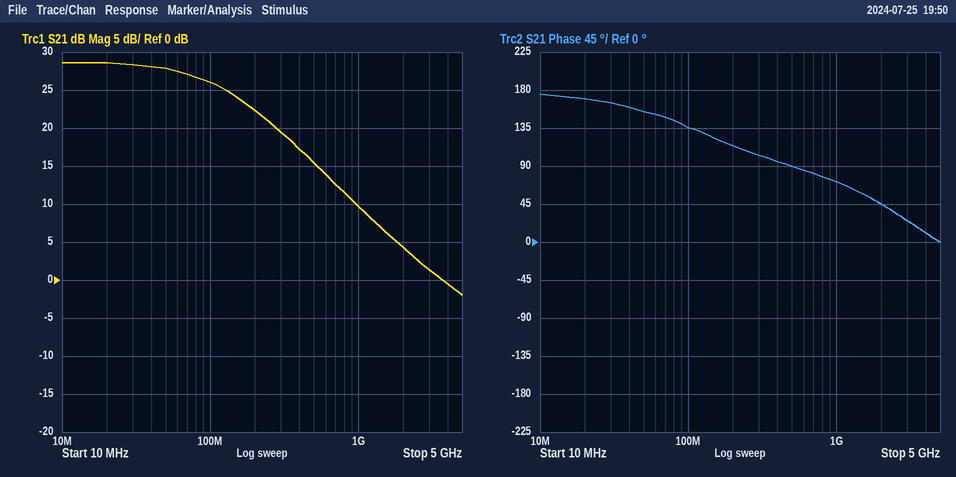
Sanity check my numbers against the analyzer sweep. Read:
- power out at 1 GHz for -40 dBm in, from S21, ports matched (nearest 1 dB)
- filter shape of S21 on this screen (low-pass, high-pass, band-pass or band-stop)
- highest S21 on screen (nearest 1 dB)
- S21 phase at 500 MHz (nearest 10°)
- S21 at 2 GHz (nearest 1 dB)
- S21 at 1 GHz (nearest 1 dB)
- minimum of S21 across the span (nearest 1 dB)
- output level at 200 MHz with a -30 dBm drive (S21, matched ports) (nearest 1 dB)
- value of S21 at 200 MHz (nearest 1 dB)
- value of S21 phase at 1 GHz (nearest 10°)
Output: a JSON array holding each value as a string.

["-30 dBm", "low-pass", "29 dB", "90°", "4 dB", "10 dB", "-2 dB", "-8 dBm", "22 dB", "70°"]
